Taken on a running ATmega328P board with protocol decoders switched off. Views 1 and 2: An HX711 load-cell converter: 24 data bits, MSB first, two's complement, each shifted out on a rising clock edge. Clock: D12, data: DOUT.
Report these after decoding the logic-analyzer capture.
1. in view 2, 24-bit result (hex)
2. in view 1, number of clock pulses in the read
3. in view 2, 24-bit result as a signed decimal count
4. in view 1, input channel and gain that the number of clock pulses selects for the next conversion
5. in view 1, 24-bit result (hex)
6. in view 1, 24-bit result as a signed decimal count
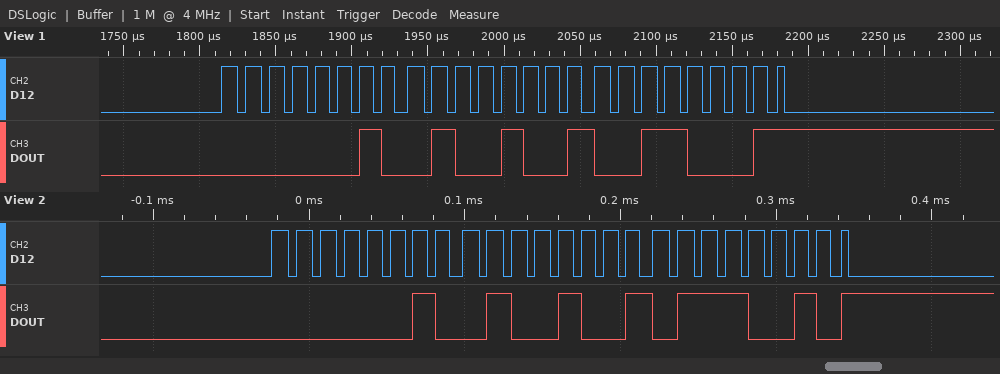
0x024972
25
149874
channel A, gain 128
0x024931
149809
